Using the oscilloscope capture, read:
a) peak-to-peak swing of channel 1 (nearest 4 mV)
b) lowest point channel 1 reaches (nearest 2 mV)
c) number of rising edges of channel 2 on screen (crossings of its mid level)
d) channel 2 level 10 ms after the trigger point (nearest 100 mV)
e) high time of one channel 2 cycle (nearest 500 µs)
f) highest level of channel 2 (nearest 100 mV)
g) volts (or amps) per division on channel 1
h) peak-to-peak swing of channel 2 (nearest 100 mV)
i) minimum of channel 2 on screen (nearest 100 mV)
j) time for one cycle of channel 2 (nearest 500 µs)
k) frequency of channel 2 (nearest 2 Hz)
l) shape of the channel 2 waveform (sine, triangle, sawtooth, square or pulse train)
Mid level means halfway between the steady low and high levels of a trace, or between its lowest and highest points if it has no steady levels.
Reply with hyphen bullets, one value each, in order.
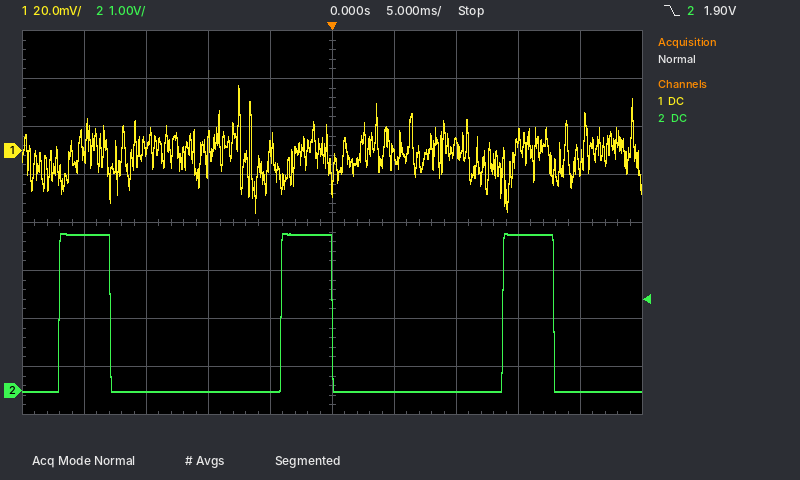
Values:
- 52 mV
- -26 mV
- 3
- 0.0 V
- 4.0 ms
- 3.3 V
- 20 mV
- 3.3 V
- 0.0 V
- 18.0 ms
- 56 Hz
- pulse train
